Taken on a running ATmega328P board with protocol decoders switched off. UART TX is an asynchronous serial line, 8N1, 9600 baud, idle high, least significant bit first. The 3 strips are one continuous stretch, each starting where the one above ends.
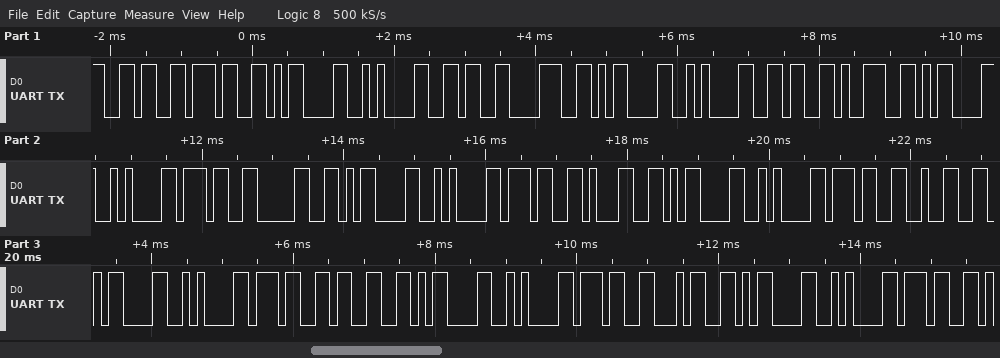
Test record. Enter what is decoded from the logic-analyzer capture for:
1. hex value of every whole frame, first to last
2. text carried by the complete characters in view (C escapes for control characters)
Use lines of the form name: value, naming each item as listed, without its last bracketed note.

hex value of every whole frame, first to last: 0x36 0x37 0x0D 0x0A 0x36 0x38 0x0D 0x0A 0x36 0x39 0x0D 0x0A 0x37 0x30 0x0D 0x0A 0x37 0x31 0x0D 0x0A 0x37 0x32 0x0D 0x0A 0x37 0x33 0x0D 0x0A 0x37 0x34 0x0D 0x0A 0x37
text carried by the complete characters in view: "67\r\n68\r\n69\r\n70\r\n71\r\n72\r\n73\r\n74\r\n7"
